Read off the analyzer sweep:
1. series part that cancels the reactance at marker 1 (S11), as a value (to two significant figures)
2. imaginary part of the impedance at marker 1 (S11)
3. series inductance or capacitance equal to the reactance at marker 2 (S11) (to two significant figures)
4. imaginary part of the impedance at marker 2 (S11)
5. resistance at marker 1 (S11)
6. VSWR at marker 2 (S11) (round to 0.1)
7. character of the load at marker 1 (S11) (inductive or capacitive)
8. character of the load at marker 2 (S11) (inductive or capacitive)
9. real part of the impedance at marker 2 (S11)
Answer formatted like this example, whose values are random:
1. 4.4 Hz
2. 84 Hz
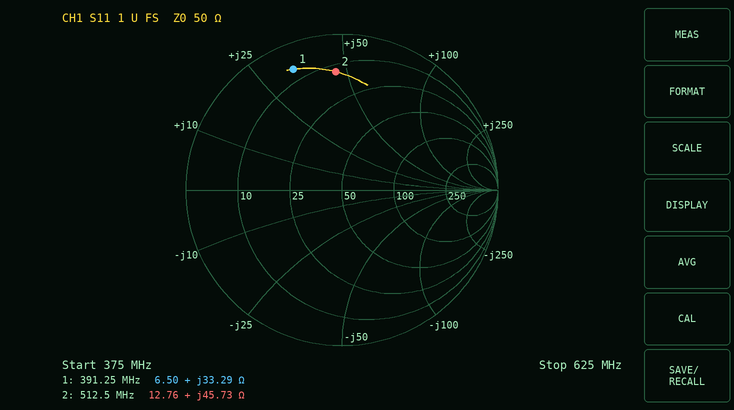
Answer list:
1. 12 pF
2. +33.29 Ω
3. 14 nH
4. +45.73 Ω
5. 6.50 Ω
6. 7.3
7. inductive
8. inductive
9. 12.76 Ω
